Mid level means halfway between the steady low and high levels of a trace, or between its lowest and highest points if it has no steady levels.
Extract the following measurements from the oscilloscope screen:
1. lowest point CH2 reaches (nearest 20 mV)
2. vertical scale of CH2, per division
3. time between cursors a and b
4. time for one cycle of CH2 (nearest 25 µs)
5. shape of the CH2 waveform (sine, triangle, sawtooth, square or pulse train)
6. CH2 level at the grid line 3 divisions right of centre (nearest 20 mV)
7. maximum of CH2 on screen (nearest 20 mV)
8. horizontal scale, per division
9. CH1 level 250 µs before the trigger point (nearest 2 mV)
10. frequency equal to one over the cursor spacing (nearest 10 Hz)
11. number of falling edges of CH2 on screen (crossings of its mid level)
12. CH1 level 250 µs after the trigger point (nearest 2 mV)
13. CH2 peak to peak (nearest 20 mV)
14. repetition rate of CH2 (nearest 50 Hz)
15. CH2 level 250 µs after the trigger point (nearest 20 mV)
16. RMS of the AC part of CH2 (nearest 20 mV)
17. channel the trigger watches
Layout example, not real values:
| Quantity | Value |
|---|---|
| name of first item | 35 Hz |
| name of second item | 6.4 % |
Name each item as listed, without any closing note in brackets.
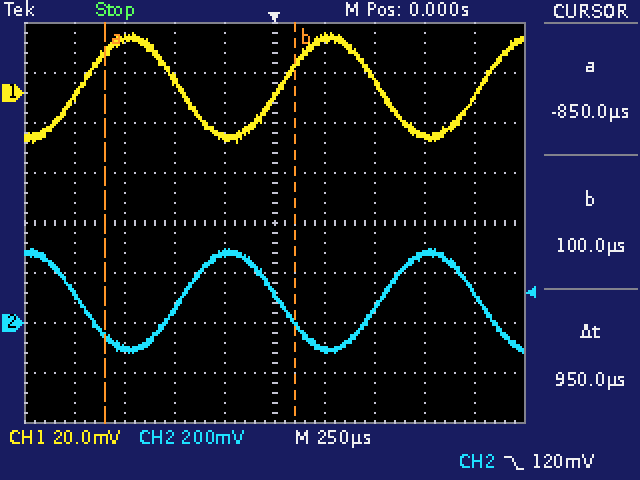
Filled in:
| Quantity | Value |
|---|---|
| lowest point CH2 reaches | -120 mV |
| vertical scale of CH2, per division | 200 mV |
| time between cursors a and b | 950 µs |
| time for one cycle of CH2 | 1.000 ms |
| shape of the CH2 waveform | sine |
| CH2 level at the grid line 3 divisions right of centre | 280 mV |
| maximum of CH2 on screen | 300 mV |
| horizontal scale, per division | 250 µs |
| CH1 level 250 µs before the trigger point | -18 mV |
| frequency equal to one over the cursor spacing | 1.05 kHz |
| number of falling edges of CH2 on screen | 3 |
| CH1 level 250 µs after the trigger point | 22 mV |
| CH2 peak to peak | 420 mV |
| repetition rate of CH2 | 1.00 kHz |
| CH2 level 250 µs after the trigger point | -100 mV |
| RMS of the AC part of CH2 | 140 mV |
| channel the trigger watches | CH2 |
